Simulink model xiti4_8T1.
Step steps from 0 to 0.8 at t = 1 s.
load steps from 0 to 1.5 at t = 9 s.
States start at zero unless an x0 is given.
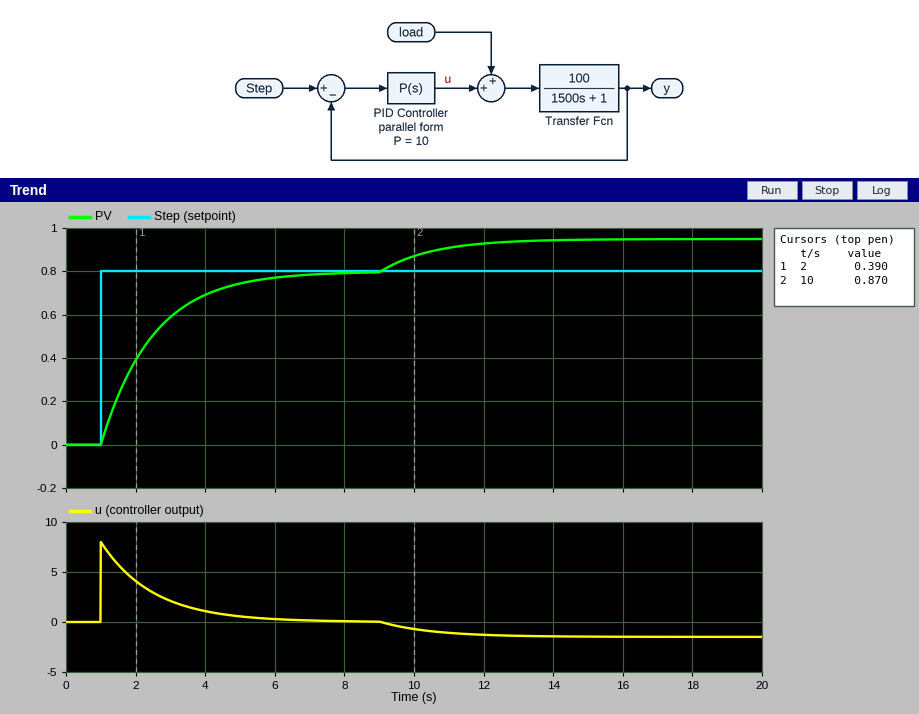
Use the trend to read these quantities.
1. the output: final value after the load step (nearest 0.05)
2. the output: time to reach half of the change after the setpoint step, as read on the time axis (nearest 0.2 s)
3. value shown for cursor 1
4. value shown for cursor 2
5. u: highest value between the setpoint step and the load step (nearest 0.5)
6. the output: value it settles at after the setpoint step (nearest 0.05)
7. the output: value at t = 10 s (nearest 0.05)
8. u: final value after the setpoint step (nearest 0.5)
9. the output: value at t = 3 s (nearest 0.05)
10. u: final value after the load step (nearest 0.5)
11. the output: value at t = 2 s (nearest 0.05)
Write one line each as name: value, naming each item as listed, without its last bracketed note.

the output: final value after the load step: 0.95
the output: time to reach half of the change after the setpoint step, as read on the time axis: 2.0 s
value shown for cursor 1: 0.390
value shown for cursor 2: 0.870
u: highest value between the setpoint step and the load step: 8.0
the output: value it settles at after the setpoint step: 0.80
the output: value at t = 10 s: 0.85
u: final value after the setpoint step: 0.0
the output: value at t = 3 s: 0.60
u: final value after the load step: -1.5
the output: value at t = 2 s: 0.40
